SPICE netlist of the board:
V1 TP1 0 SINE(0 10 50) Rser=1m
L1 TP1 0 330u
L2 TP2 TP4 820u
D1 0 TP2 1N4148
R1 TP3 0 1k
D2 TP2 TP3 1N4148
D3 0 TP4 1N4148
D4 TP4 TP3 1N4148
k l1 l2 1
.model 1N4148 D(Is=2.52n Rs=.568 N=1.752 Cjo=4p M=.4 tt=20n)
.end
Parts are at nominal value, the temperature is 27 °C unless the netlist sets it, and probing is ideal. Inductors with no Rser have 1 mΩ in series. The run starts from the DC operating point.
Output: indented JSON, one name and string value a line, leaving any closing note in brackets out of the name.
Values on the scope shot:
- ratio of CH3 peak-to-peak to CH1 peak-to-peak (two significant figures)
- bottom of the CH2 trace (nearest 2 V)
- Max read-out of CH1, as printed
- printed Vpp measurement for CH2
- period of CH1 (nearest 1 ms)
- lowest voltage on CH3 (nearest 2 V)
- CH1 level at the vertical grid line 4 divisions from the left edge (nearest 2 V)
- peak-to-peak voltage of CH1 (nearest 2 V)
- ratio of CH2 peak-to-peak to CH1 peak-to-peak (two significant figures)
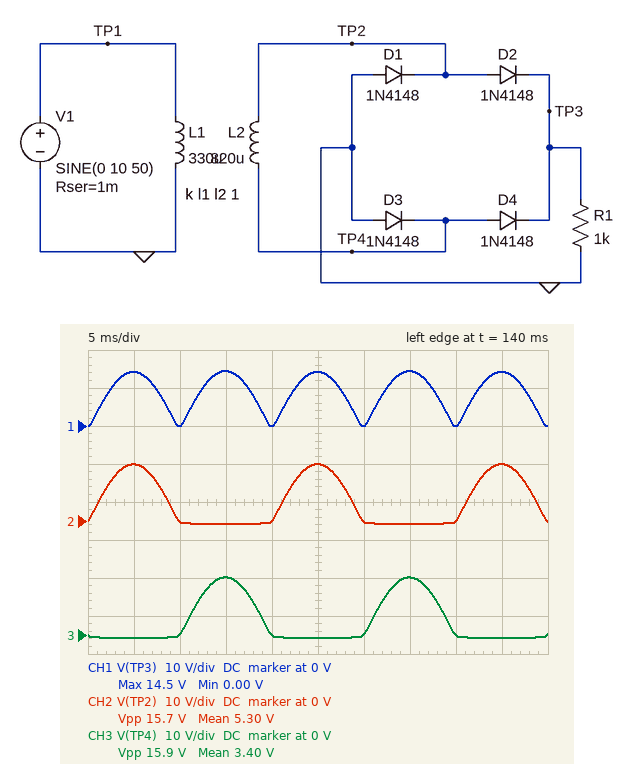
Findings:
{
  "ratio of CH3 peak-to-peak to CH1 peak-to-peak": "1.1",
  "bottom of the CH2 trace": "0 V",
  "Max read-out of CH1, as printed": "14.5 V",
  "printed Vpp measurement for CH2": "15.7 V",
  "period of CH1": "10 ms",
  "lowest voltage on CH3": "0 V",
  "CH1 level at the vertical grid line 4 divisions from the left edge": "0 V",
  "peak-to-peak voltage of CH1": "14 V",
  "ratio of CH2 peak-to-peak to CH1 peak-to-peak": "1.1"
}
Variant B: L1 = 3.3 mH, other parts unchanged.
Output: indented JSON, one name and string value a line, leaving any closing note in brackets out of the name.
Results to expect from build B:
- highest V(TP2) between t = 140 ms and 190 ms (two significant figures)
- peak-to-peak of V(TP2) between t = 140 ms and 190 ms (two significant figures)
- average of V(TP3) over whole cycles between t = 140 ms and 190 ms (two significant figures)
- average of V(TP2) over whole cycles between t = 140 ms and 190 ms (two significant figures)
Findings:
{
  "highest V(TP2) between t = 140 ms and 190 ms": "4.3 V",
  "peak-to-peak of V(TP2) between t = 140 ms and 190 ms": "5.0 V",
  "average of V(TP3) over whole cycles between t = 140 ms and 190 ms": "2.0 V",
  "average of V(TP2) over whole cycles between t = 140 ms and 190 ms": "1.0 V"
}
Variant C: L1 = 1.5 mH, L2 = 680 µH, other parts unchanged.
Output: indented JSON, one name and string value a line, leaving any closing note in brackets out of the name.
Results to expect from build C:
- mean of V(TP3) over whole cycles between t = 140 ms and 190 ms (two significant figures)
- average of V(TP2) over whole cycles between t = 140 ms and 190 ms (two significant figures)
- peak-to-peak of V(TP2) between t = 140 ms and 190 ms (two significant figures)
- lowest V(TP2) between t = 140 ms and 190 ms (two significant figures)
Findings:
{
  "mean of V(TP3) over whole cycles between t = 140 ms and 190 ms": "3.1 V",
  "average of V(TP2) over whole cycles between t = 140 ms and 190 ms": "1.5 V",
  "peak-to-peak of V(TP2) between t = 140 ms and 190 ms": "6.7 V",
  "lowest V(TP2) between t = 140 ms and 190 ms": "-660 mV"
}
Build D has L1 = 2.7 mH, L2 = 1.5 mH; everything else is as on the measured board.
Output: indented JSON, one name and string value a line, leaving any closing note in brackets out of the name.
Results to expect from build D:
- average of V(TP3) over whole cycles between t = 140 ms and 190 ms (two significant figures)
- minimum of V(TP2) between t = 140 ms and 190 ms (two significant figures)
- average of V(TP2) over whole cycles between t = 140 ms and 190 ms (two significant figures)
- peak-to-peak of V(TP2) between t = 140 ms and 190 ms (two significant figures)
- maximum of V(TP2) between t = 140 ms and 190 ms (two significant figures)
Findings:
{
  "average of V(TP3) over whole cycles between t = 140 ms and 190 ms": "3.5 V",
  "minimum of V(TP2) between t = 140 ms and 190 ms": "-670 mV",
  "average of V(TP2) over whole cycles between t = 140 ms and 190 ms": "1.8 V",
  "peak-to-peak of V(TP2) between t = 140 ms and 190 ms": "7.4 V",
  "maximum of V(TP2) between t = 140 ms and 190 ms": "6.8 V"
}
